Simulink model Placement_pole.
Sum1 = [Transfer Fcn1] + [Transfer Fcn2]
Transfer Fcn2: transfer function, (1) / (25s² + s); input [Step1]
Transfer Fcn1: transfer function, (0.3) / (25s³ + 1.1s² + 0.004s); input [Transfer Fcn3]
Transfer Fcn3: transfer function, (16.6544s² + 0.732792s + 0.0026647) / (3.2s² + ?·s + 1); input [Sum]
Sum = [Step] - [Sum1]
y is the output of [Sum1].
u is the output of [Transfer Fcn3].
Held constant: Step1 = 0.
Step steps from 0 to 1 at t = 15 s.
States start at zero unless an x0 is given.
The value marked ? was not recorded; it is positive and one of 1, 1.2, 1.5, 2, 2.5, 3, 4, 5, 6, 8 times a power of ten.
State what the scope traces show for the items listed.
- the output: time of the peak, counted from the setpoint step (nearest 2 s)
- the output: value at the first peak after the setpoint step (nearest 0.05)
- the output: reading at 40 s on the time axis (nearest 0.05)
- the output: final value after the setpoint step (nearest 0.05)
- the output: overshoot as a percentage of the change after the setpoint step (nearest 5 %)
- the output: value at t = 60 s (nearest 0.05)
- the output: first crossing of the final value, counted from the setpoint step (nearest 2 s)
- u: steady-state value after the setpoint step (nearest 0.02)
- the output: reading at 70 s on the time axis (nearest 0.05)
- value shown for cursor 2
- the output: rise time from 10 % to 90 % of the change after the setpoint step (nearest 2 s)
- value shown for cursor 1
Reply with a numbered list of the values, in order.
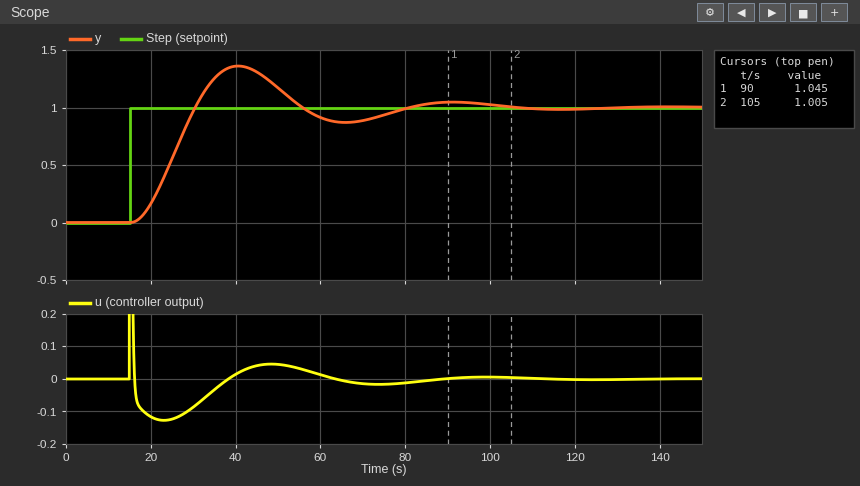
1. 26 s
2. 1.35
3. 1.35
4. 1.00
5. 35 %
6. 0.90
7. 16 s
8. 0.00
9. 0.90
10. 1.005
11. 10 s
12. 1.045
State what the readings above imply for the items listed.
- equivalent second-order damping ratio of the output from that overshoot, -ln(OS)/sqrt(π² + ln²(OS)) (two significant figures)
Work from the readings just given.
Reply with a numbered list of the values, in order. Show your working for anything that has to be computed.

1. ln(0.35) = -1.050; 1.050 / sqrt(9.870 + 1.102) = 0.32
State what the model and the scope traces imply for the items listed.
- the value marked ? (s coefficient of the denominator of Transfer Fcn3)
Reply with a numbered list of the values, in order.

1. 12
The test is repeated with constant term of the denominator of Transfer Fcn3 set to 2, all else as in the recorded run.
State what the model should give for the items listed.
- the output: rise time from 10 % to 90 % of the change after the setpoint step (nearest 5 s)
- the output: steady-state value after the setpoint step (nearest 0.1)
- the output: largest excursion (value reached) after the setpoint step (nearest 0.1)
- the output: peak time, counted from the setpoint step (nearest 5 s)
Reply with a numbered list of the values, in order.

1. 15 s
2. 1.0
3. 1.1
4. 30 s
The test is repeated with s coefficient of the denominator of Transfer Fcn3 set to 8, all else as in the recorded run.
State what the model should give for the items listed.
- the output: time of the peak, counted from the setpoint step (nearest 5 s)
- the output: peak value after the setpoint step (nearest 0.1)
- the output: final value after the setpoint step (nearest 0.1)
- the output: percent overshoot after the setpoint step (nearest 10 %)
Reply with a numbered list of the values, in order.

1. 20 s
2. 1.3
3. 1.0
4. 30 %
